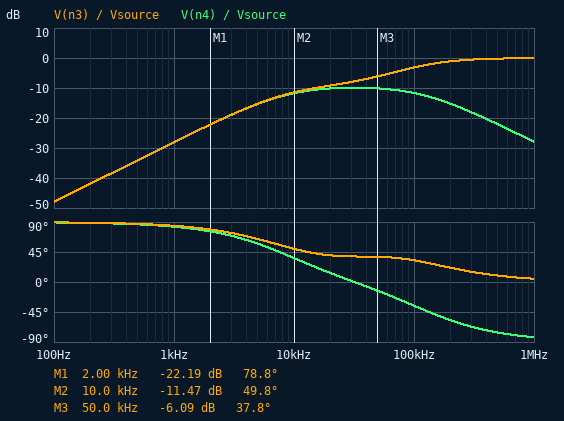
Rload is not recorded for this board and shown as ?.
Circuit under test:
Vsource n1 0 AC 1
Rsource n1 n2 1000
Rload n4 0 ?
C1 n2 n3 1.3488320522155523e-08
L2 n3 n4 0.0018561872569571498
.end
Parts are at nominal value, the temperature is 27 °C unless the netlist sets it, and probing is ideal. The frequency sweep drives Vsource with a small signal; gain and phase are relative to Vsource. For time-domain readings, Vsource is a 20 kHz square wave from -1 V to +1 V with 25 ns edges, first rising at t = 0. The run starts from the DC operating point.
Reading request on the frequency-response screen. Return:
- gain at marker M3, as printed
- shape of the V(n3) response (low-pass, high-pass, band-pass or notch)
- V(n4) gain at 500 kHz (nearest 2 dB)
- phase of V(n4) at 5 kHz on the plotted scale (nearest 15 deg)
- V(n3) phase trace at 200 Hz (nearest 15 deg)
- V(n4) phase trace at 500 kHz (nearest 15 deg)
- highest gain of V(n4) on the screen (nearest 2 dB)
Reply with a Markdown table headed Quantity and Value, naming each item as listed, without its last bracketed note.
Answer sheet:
| Quantity | Value |
|---|---|
| gain at marker M3, as printed | -6.09 dB |
| shape of the V(n3) response | high-pass |
| V(n4) gain at 500 kHz | -22 dB |
| phase of V(n4) at 5 kHz on the plotted scale | 60 deg |
| V(n3) phase trace at 200 Hz | 90 deg |
| V(n4) phase trace at 500 kHz | -75 deg |
| highest gain of V(n4) on the screen | -10 dB |
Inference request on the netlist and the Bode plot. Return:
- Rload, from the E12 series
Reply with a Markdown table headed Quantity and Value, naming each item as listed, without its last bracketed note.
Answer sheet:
| Quantity | Value |
|---|---|
| Rload, from the E12 series | 470 Ω |
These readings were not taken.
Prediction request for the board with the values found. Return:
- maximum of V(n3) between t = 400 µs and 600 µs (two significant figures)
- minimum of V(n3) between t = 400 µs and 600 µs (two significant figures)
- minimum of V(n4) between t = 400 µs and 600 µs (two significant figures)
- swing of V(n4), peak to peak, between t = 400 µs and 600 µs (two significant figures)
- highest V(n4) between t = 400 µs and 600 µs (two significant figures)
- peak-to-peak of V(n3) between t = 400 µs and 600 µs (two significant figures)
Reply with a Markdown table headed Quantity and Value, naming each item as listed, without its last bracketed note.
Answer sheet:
| Quantity | Value |
|---|---|
| maximum of V(n3) between t = 400 µs and 600 µs | 1.9 V |
| minimum of V(n3) between t = 400 µs and 600 µs | -1.9 V |
| minimum of V(n4) between t = 400 µs and 600 µs | -440 mV |
| swing of V(n4), peak to peak, between t = 400 µs and 600 µs | 870 mV |
| highest V(n4) between t = 400 µs and 600 µs | 440 mV |
| peak-to-peak of V(n3) between t = 400 µs and 600 µs | 3.7 V |
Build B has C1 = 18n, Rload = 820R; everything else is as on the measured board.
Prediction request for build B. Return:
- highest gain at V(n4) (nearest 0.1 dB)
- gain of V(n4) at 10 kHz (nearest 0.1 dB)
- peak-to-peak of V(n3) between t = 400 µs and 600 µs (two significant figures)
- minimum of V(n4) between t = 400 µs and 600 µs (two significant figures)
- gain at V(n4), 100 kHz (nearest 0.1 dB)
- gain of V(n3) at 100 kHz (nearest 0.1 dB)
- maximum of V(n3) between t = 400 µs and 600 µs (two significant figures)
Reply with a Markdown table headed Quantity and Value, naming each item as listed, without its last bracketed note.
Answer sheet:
| Quantity | Value |
|---|---|
| highest gain at V(n4) | -6.9 dB |
| gain of V(n4) at 10 kHz | -7.6 dB |
| peak-to-peak of V(n3) between t = 400 µs and 600 µs | 3.4 V |
| minimum of V(n4) between t = 400 µs and 600 µs | -560 mV |
| gain at V(n4), 100 kHz | -8.2 dB |
| gain of V(n3) at 100 kHz | -3.4 dB |
| maximum of V(n3) between t = 400 µs and 600 µs | 1.7 V |
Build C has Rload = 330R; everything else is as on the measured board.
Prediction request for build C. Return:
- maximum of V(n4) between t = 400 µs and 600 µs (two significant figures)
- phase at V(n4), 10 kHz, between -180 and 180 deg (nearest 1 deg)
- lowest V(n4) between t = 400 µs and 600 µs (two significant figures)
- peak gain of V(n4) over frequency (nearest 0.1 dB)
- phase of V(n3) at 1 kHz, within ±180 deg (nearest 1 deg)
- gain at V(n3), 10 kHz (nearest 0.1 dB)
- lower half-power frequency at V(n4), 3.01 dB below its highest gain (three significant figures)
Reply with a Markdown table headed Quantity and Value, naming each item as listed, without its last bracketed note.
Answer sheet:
| Quantity | Value |
|---|---|
| maximum of V(n4) between t = 400 µs and 600 µs | 340 mV |
| phase at V(n4), 10 kHz, between -180 and 180 deg | 39 deg |
| lowest V(n4) between t = 400 µs and 600 µs | -340 mV |
| peak gain of V(n4) over frequency | -12.1 dB |
| phase of V(n3) at 1 kHz, within ±180 deg | 86 deg |
| gain at V(n3), 10 kHz | -13.7 dB |
| lower half-power frequency at V(n4), 3.01 dB below its highest gain | 8.27 kHz |
